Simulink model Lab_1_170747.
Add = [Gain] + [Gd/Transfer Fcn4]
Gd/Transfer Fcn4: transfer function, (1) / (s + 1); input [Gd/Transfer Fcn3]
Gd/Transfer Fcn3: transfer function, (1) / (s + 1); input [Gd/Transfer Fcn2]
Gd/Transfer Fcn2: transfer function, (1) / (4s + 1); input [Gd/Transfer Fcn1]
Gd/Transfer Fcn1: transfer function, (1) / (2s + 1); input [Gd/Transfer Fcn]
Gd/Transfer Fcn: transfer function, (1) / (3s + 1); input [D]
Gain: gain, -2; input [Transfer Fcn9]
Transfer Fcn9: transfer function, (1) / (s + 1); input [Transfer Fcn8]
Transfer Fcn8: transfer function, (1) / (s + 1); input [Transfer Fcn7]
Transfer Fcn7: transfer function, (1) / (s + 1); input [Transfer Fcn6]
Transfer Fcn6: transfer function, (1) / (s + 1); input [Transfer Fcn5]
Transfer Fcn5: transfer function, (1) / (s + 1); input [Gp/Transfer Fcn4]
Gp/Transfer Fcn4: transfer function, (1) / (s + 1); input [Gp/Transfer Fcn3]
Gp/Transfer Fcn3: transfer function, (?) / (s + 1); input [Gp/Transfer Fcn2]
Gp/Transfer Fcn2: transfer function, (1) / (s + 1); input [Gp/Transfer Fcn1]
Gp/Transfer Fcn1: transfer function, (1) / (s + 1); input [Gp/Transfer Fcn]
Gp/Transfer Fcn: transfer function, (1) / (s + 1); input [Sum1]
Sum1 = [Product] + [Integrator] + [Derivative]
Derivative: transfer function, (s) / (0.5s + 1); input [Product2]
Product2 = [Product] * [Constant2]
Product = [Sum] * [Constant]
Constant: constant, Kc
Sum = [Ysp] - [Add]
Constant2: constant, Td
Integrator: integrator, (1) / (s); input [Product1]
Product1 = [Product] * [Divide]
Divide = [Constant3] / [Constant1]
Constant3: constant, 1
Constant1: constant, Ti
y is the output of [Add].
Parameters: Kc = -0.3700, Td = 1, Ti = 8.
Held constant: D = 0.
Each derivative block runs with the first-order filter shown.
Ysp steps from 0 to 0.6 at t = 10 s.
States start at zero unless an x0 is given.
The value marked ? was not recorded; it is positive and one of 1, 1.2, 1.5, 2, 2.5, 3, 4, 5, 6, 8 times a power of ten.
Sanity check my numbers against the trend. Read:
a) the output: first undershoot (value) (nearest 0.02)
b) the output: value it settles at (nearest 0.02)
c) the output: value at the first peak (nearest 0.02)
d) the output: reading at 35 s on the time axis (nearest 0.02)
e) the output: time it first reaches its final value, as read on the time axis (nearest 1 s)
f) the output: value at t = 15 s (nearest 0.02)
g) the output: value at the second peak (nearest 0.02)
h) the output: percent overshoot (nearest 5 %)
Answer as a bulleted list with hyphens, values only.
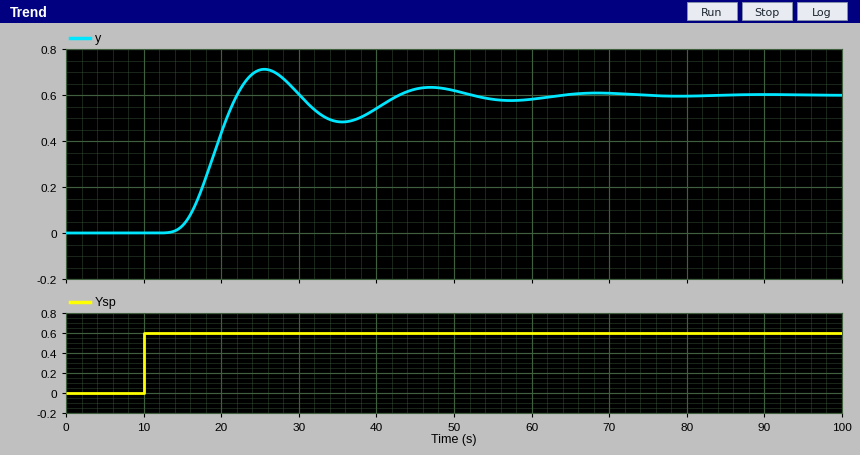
- 0.48
- 0.60
- 0.72
- 0.48
- 22 s
- 0.04
- 0.64
- 20 %
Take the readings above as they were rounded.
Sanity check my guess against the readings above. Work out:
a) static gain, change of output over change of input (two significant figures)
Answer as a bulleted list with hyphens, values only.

- 1.0
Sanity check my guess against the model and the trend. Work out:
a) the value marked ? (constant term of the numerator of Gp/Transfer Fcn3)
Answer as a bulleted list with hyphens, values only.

- 1.2
